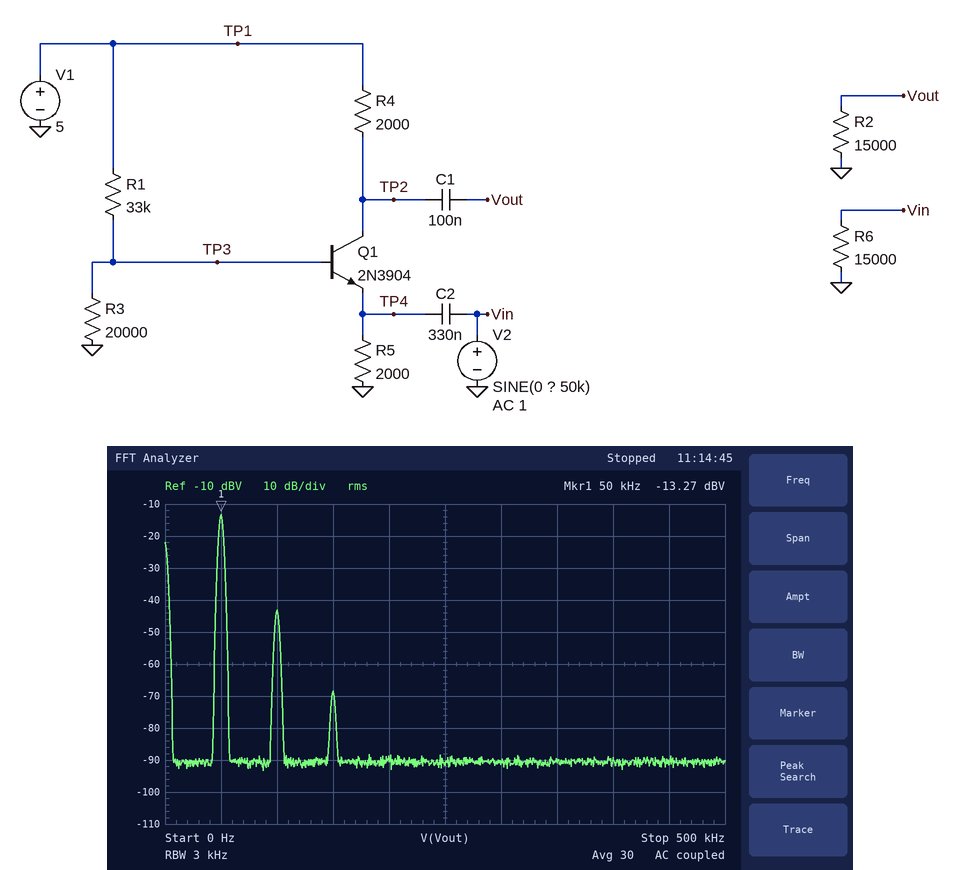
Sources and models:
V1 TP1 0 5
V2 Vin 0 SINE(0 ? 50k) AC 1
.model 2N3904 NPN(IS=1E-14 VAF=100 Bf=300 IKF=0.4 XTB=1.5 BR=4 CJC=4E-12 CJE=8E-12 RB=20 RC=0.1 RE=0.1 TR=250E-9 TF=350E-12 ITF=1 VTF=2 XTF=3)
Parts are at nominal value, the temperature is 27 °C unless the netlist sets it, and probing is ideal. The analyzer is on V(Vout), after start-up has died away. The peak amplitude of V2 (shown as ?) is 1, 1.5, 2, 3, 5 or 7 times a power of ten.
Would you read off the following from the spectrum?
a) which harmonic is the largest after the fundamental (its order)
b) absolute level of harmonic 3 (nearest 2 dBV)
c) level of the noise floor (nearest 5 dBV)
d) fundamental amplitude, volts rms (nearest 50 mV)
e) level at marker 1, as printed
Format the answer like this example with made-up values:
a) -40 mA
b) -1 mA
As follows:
a) 2
b) -68 dBV
c) -90 dBV
d) 200 mV
e) -13.27 dBV
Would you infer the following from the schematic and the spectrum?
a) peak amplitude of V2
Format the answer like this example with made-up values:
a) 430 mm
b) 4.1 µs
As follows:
a) 15 mV
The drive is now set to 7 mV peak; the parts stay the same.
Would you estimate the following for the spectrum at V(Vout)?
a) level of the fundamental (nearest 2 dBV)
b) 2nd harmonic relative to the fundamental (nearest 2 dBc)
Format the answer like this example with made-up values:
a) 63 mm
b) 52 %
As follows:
a) -20 dBV
b) -36 dBc
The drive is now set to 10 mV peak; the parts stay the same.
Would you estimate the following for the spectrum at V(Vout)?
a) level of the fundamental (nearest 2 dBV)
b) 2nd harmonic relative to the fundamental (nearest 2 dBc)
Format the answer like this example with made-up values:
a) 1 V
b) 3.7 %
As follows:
a) -16 dBV
b) -34 dBc
